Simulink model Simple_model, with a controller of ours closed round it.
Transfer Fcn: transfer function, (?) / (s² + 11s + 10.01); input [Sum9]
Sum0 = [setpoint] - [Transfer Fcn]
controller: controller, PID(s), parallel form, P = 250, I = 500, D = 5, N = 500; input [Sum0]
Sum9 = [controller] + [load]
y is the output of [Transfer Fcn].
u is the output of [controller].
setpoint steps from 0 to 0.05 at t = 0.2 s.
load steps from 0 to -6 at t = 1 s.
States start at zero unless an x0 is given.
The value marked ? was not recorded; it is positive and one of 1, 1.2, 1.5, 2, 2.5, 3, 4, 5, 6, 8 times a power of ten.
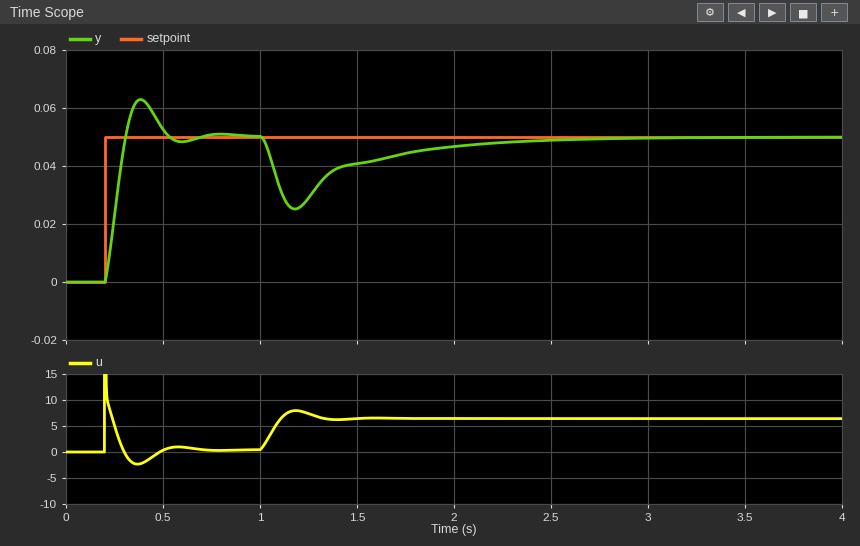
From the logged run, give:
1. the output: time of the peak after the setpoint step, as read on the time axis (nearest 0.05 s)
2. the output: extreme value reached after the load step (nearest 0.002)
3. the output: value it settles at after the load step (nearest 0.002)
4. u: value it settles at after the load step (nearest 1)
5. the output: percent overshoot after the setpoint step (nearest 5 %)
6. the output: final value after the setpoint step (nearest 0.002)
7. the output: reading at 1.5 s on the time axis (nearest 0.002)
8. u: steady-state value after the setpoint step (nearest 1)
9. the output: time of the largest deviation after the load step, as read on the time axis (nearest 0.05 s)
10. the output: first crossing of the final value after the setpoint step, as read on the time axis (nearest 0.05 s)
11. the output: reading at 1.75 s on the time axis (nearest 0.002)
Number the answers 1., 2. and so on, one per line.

1. 0.40 s
2. 0.026
3. 0.050
4. 6
5. 25 %
6. 0.050
7. 0.040
8. 0
9. 1.20 s
10. 0.30 s
11. 0.044
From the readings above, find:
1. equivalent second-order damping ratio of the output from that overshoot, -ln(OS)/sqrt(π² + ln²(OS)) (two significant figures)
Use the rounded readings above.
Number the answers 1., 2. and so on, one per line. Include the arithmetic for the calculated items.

1. ln(0.25) = -1.386; 1.386 / sqrt(9.870 + 1.922) = 0.40
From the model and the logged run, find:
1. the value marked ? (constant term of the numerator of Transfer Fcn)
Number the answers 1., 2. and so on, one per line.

1. 1.2
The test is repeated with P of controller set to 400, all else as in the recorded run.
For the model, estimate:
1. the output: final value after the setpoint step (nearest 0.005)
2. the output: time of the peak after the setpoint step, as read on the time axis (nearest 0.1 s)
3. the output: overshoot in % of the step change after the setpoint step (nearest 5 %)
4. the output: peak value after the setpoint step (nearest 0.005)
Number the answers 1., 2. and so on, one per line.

1. 0.050
2. 0.3 s
3. 30 %
4. 0.065
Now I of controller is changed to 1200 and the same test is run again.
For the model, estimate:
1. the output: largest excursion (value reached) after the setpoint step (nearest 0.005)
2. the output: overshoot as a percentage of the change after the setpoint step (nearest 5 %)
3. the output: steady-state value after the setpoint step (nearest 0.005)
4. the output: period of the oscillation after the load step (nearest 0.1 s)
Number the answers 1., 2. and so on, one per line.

1. 0.070
2. 40 %
3. 0.050
4. 0.4 s
